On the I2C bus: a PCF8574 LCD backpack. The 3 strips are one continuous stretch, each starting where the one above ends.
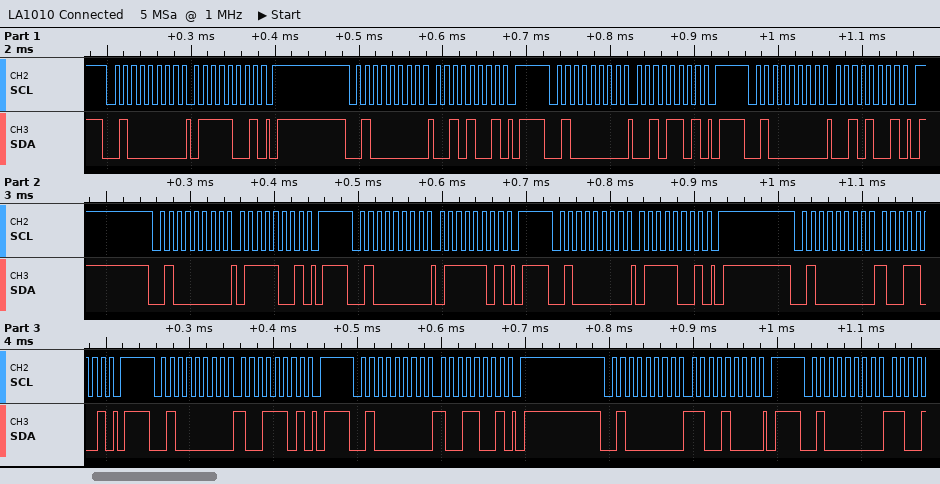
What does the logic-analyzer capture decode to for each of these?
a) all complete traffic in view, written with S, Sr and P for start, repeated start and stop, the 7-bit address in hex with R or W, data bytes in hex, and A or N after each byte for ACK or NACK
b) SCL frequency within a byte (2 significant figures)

S 20W A 79 A P S 20W A 29 A P S 20W A 2D A P S 20W A 29 A P S 20W A 79 A P S 20W A 7D A P S 20W A 79 A P S 20W A 99 A P S 20W A 9D A P S 20W A 99 A P S 20W A C8 A P S 20W A
100 kHz
